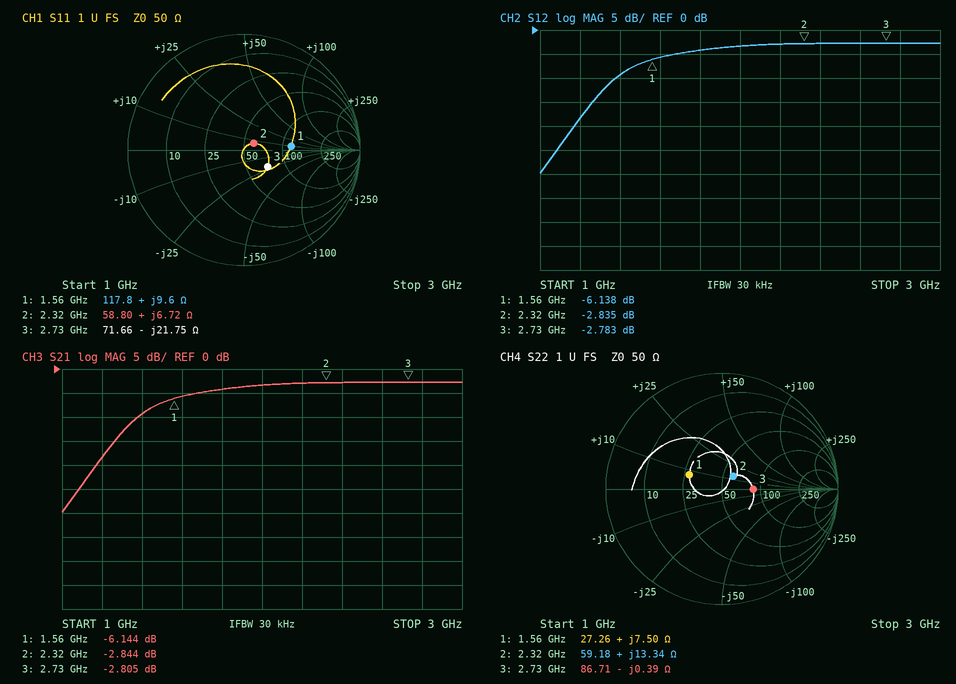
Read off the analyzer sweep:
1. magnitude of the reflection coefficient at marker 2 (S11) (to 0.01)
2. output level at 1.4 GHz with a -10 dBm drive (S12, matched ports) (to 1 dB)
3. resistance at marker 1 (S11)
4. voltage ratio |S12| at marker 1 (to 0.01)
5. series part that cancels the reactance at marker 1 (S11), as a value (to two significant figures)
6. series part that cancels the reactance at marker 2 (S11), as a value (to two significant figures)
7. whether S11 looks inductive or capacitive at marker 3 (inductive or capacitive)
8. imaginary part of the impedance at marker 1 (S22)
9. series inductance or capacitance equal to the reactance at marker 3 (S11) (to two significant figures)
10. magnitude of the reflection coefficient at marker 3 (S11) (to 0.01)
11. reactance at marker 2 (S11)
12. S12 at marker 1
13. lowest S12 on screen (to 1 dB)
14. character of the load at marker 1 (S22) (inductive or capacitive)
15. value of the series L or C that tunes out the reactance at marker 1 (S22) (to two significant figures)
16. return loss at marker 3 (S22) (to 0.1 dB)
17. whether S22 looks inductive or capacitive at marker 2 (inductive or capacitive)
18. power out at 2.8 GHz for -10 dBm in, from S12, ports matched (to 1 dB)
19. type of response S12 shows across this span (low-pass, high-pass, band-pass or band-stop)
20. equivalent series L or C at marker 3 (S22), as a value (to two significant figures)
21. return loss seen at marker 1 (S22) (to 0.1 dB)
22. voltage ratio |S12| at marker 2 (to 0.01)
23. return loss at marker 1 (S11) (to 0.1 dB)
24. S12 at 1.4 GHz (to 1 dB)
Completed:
0.10
-19 dBm
117.8 Ω
0.49
11 pF
10 pF
capacitive
+7.50 Ω
2.7 pF
0.25
+6.72 Ω
-6.138 dB
-30 dB
inductive
14 pF
11.4 dB
inductive
-13 dBm
high-pass
150 pF
10.2 dB
0.72
7.8 dB
-9 dB
